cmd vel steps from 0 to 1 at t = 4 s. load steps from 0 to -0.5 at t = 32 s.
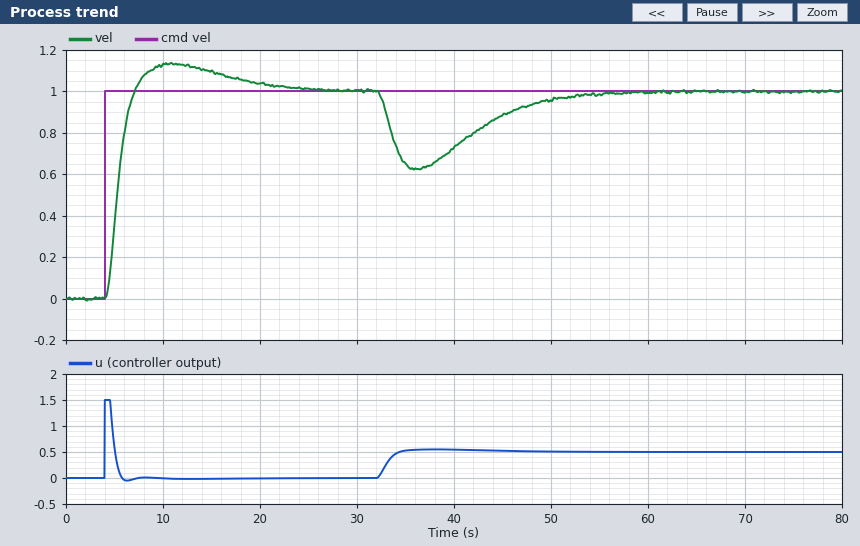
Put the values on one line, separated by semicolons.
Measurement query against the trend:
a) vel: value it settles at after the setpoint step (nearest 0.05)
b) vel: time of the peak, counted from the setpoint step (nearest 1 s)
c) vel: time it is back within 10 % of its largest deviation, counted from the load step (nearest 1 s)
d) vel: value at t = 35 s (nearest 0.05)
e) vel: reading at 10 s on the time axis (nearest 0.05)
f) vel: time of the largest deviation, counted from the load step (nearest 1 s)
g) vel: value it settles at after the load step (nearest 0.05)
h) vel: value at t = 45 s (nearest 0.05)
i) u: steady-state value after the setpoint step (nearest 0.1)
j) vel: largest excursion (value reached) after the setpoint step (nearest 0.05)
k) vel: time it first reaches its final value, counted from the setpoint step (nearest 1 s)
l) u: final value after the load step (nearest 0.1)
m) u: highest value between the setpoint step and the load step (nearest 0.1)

1.00; 7 s; 18 s; 0.65; 1.15; 4 s; 1.00; 0.90; 0.0; 1.15; 3 s; 0.5; 1.5
